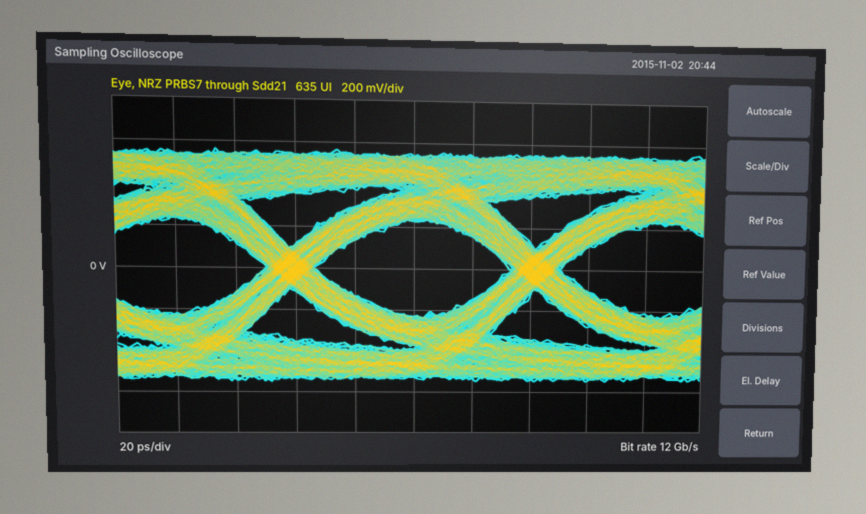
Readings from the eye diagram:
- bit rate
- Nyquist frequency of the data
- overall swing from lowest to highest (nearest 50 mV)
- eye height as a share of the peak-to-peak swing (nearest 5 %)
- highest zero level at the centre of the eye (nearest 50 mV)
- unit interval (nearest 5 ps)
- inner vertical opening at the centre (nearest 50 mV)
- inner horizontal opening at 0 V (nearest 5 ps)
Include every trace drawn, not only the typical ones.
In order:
12 Gb/s
6 GHz
1.10 V
40 %
-250 mV
85 ps
450 mV
65 ps
